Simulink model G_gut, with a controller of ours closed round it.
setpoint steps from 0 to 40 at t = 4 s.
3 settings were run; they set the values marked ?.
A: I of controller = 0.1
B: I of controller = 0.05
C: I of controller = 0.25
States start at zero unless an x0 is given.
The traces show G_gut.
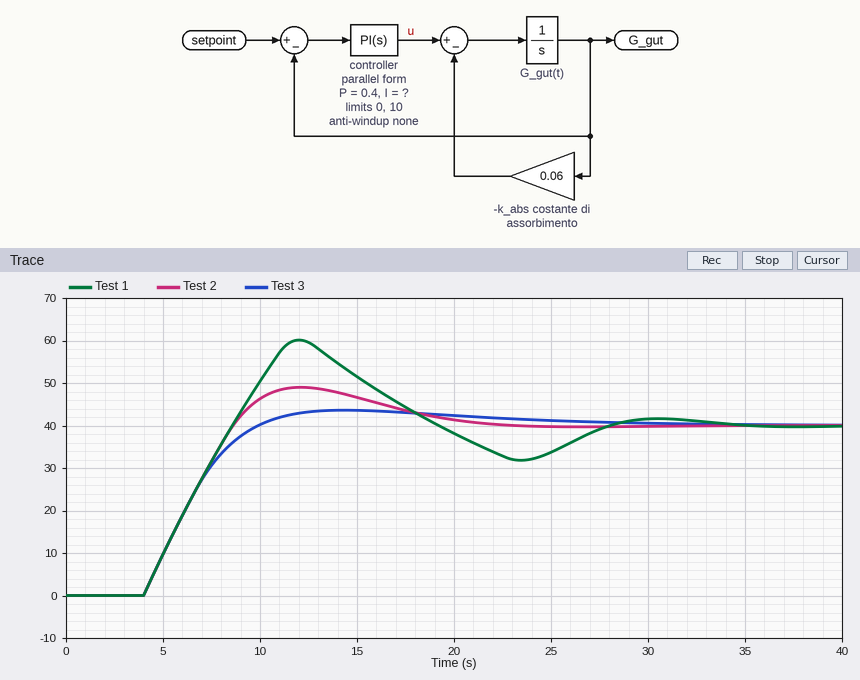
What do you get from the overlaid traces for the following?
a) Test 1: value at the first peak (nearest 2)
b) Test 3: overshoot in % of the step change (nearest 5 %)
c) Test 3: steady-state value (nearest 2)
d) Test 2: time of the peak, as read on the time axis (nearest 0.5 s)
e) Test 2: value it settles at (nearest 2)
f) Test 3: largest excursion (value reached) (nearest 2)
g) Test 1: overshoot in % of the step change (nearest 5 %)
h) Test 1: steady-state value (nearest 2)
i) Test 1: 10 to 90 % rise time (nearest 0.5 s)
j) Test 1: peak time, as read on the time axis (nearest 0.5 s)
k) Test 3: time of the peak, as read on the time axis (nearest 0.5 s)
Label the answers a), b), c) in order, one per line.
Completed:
a) 60
b) 10 %
c) 40
d) 12.0 s
e) 40
f) 44
g) 50 %
h) 40
i) 3.5 s
j) 12.0 s
k) 14.5 s
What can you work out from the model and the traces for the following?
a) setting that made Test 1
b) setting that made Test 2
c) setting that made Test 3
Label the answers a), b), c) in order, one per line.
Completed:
a) C
b) A
c) B
